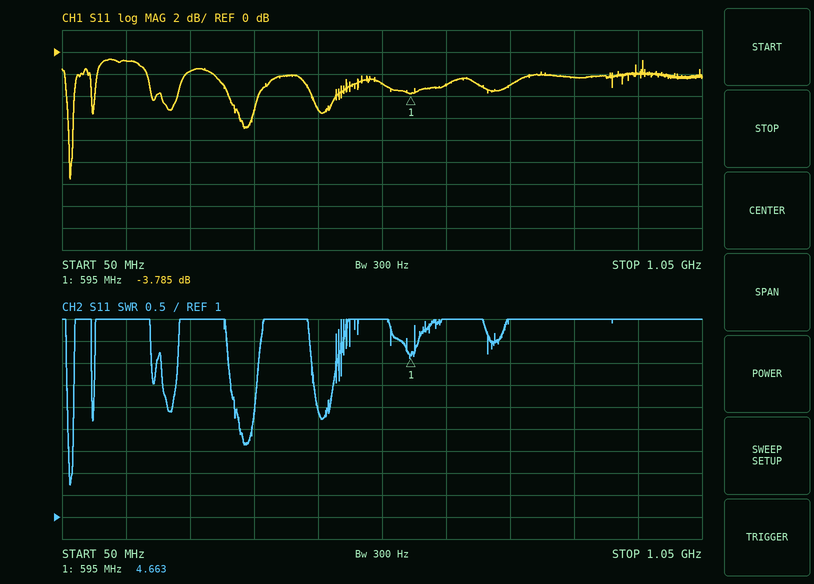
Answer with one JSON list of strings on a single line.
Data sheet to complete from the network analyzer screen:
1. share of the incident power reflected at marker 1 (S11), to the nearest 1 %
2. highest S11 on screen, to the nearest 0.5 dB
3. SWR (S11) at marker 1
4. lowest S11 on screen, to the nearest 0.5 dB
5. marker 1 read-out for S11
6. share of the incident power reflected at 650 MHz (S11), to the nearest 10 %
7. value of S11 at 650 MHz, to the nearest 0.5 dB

["42 %", "-0.5 dB", "4.663", "-11.5 dB", "-3.785 dB", "50 %", "-3.0 dB"]
